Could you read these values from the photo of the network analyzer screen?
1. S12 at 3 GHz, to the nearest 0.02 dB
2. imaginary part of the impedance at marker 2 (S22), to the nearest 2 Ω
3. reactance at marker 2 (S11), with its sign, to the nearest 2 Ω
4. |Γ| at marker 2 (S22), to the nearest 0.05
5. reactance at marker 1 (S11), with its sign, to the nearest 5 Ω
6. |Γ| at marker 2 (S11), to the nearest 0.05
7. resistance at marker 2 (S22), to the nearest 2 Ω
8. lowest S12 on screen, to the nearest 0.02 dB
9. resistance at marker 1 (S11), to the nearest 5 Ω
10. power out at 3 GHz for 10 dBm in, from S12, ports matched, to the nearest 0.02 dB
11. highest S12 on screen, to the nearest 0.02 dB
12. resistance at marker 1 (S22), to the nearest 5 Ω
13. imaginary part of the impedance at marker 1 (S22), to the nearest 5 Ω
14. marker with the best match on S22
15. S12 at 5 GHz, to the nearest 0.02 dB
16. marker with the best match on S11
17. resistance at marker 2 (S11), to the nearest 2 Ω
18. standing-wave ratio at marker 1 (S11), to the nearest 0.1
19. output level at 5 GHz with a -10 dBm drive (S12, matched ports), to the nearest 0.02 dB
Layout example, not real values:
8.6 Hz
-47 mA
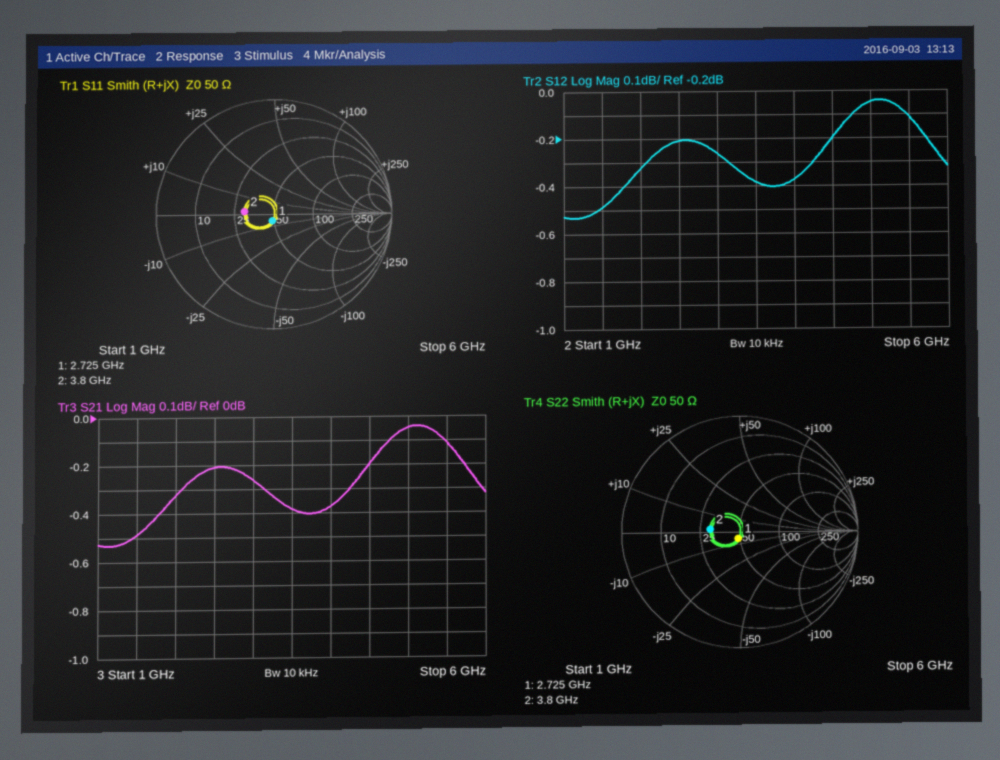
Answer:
-0.26 dB
+2 Ω
+2 Ω
0.25
-5 Ω
0.25
30 Ω
-0.54 dB
50 Ω
9.74 dBm
-0.04 dB
50 Ω
-5 Ω
marker 1
-0.04 dB
marker 1
30 Ω
1.1
-10.04 dBm
